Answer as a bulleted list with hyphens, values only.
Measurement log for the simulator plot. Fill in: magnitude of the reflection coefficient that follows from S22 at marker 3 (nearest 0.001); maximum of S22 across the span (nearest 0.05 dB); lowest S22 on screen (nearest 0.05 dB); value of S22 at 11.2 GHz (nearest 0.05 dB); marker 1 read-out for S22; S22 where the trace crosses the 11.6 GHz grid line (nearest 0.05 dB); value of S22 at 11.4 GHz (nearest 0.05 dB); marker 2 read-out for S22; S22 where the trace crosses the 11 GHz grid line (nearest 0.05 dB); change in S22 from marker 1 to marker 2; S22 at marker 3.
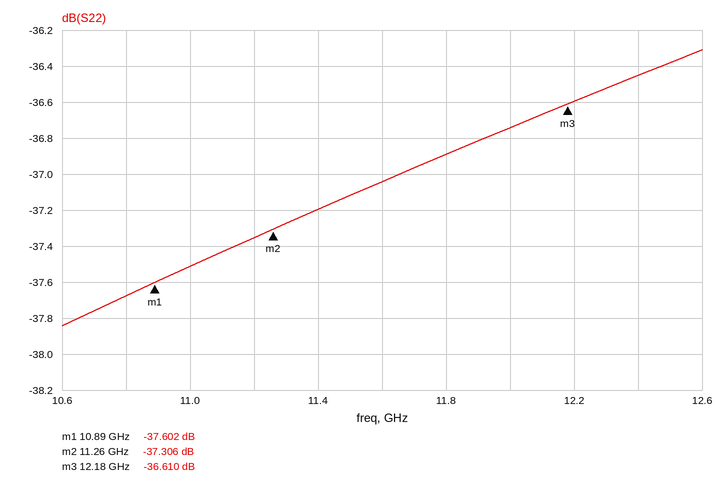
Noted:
- 0.015
- -36.30 dB
- -37.85 dB
- -37.35 dB
- -37.602 dB
- -37.05 dB
- -37.20 dB
- -37.306 dB
- -37.50 dB
- 0.296 dB
- -36.610 dB
